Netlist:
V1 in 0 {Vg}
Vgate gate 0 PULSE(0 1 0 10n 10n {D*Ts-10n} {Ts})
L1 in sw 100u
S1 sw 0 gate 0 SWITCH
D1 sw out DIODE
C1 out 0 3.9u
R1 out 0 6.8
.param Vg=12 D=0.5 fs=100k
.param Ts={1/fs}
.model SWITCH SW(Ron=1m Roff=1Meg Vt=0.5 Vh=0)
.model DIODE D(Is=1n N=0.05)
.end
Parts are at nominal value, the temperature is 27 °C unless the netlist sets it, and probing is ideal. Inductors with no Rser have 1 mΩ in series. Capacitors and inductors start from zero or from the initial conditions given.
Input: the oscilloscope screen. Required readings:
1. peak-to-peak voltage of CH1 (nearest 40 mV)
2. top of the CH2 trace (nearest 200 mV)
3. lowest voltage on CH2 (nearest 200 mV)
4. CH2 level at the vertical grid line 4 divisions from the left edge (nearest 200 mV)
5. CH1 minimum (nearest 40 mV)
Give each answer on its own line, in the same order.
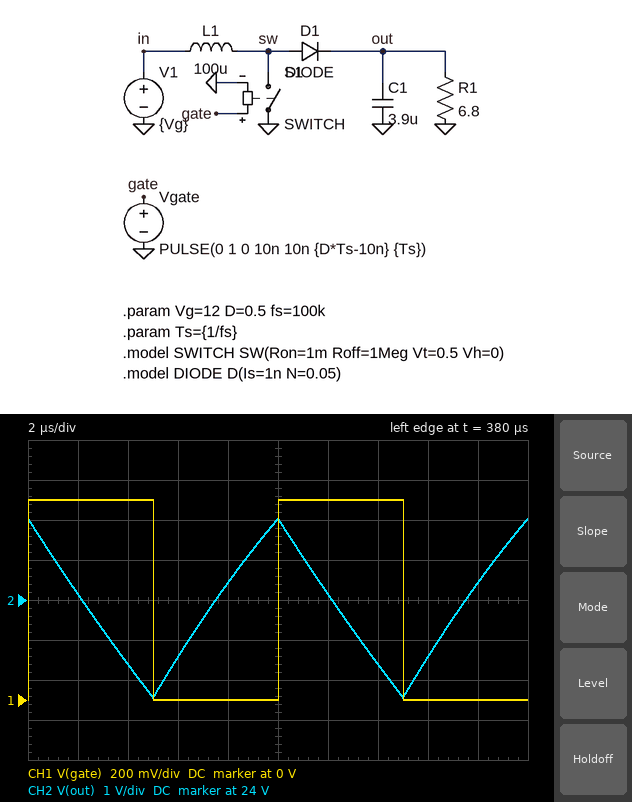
1.00 V
26.0 V
21.6 V
24.4 V
0 V
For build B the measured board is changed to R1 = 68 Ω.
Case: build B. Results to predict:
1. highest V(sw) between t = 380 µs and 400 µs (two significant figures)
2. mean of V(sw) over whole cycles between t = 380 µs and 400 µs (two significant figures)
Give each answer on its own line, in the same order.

22 V
11 V
